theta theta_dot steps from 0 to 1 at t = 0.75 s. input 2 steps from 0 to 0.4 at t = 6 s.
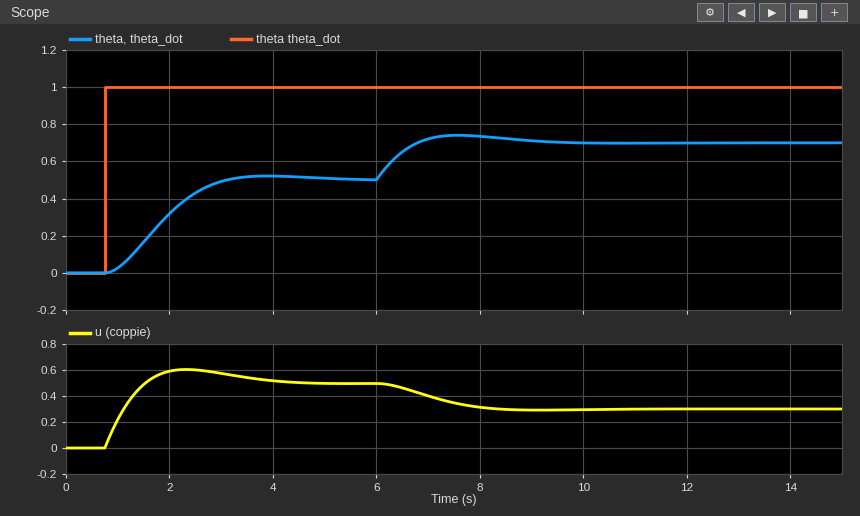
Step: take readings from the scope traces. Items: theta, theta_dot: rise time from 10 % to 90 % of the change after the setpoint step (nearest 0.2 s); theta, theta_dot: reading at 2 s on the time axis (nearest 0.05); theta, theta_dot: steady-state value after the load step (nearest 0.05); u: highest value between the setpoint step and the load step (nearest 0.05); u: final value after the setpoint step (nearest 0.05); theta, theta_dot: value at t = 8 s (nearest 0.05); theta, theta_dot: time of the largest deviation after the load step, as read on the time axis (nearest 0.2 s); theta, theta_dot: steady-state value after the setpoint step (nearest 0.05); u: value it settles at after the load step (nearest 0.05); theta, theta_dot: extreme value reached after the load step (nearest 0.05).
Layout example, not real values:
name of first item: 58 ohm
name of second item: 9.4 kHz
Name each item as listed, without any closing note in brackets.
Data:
theta, theta_dot: rise time from 10 % to 90 % of the change after the setpoint step: 1.6 s
theta, theta_dot: reading at 2 s on the time axis: 0.30
theta, theta_dot: steady-state value after the load step: 0.70
u: highest value between the setpoint step and the load step: 0.60
u: final value after the setpoint step: 0.50
theta, theta_dot: value at t = 8 s: 0.75
theta, theta_dot: time of the largest deviation after the load step, as read on the time axis: 7.6 s
theta, theta_dot: steady-state value after the setpoint step: 0.50
u: value it settles at after the load step: 0.30
theta, theta_dot: extreme value reached after the load step: 0.75
